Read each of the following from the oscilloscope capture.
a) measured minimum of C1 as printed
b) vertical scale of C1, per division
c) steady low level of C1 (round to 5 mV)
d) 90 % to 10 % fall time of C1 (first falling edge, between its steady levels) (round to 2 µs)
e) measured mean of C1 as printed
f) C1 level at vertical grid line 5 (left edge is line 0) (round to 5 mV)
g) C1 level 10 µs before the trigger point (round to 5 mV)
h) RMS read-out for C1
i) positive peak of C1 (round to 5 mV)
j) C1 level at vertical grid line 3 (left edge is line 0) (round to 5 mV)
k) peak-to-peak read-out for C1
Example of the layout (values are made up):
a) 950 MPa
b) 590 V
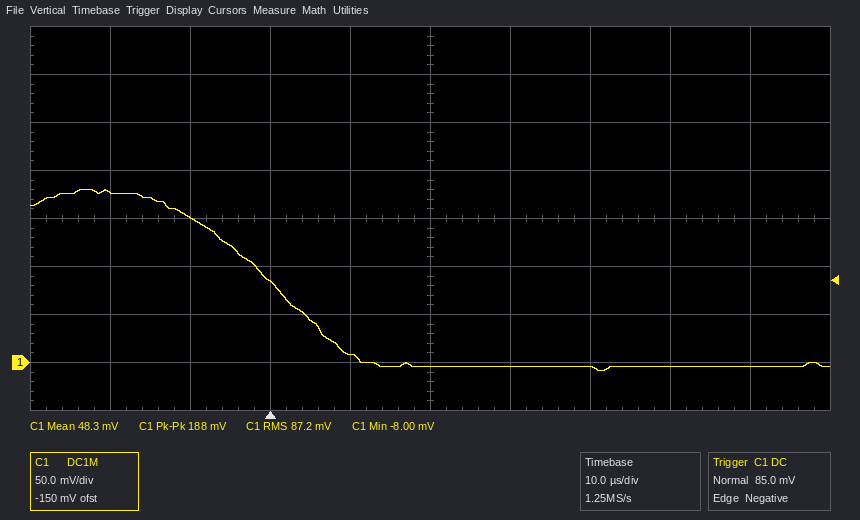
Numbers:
a) -8.00 mV
b) 50 mV
c) -5 mV
d) 20 µs
e) 48.3 mV
f) -5 mV
g) 150 mV
h) 87.2 mV
i) 180 mV
j) 85 mV
k) 188 mV
